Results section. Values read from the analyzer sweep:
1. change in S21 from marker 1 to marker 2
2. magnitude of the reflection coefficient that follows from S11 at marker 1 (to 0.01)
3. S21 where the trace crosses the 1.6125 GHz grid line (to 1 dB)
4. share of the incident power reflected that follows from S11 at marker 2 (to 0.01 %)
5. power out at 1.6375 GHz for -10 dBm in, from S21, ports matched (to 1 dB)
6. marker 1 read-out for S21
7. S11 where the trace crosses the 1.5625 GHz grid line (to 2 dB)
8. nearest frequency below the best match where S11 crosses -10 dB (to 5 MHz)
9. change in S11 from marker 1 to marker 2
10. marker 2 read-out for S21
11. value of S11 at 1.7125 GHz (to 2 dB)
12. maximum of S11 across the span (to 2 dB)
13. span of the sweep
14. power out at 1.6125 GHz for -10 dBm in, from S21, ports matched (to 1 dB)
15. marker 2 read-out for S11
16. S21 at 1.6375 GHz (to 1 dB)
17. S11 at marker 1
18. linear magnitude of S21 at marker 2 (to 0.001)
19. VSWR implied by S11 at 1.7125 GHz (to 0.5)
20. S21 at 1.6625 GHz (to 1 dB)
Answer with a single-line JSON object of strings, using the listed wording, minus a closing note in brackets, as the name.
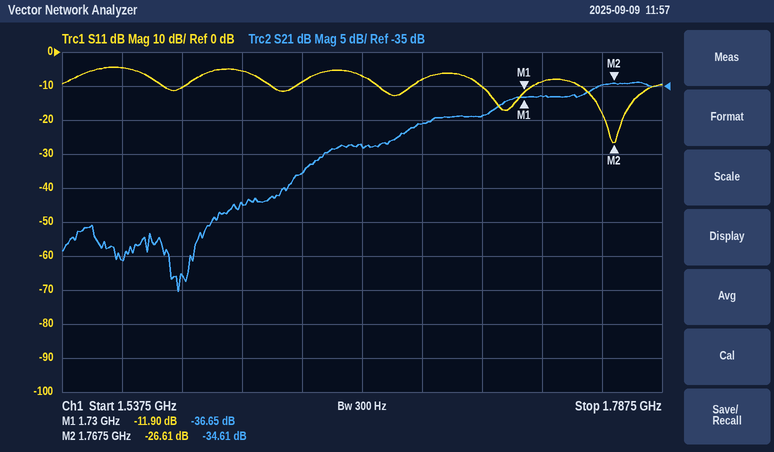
{"change in S21 from marker 1 to marker 2": "2.04 dB", "magnitude of the reflection coefficient that follows from S11 at marker 1": "0.25", "S21 where the trace crosses the 1.6125 GHz grid line": "-52 dB", "share of the incident power reflected that follows from S11 at marker 2": "0.22 %", "power out at 1.6375 GHz for -10 dBm in, from S21, ports matched": "-58 dBm", "marker 1 read-out for S21": "-36.65 dB", "S11 where the trace crosses the 1.5625 GHz grid line": "-4 dB", "nearest frequency below the best match where S11 crosses -10 dB": "1.755 GHz", "change in S11 from marker 1 to marker 2": "-14.71 dB", "marker 2 read-out for S21": "-34.61 dB", "value of S11 at 1.7125 GHz": "-10 dB", "maximum of S11 across the span": "-4 dB", "span of the sweep": "250 MHz", "power out at 1.6125 GHz for -10 dBm in, from S21, ports matched": "-62 dBm", "marker 2 read-out for S11": "-26.61 dB", "S21 at 1.6375 GHz": "-48 dB", "S11 at marker 1": "-11.90 dB", "linear magnitude of S21 at marker 2": "0.019", "VSWR implied by S11 at 1.7125 GHz": "2.0", "S21 at 1.6625 GHz": "-44 dB"}
